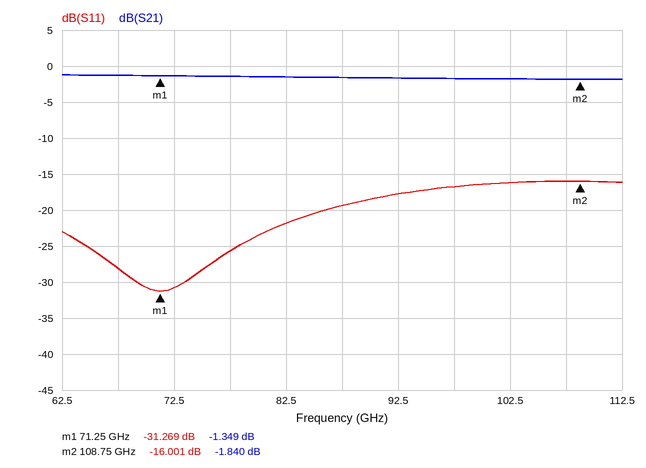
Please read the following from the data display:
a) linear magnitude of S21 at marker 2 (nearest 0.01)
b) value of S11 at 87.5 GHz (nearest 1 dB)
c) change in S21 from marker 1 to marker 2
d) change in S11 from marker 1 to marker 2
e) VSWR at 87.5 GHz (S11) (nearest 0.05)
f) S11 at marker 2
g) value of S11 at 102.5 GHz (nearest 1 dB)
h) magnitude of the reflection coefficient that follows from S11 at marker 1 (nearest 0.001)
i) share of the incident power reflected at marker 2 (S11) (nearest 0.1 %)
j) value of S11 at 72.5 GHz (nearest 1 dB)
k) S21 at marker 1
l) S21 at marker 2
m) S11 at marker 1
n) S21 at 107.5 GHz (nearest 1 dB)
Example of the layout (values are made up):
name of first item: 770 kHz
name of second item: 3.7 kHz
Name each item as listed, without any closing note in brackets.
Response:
linear magnitude of S21 at marker 2: 0.81
value of S11 at 87.5 GHz: -19 dB
change in S21 from marker 1 to marker 2: -0.491 dB
change in S11 from marker 1 to marker 2: 15.268 dB
VSWR at 87.5 GHz (S11): 1.25
S11 at marker 2: -16.001 dB
value of S11 at 102.5 GHz: -16 dB
magnitude of the reflection coefficient that follows from S11 at marker 1: 0.027
share of the incident power reflected at marker 2 (S11): 2.5 %
value of S11 at 72.5 GHz: -31 dB
S21 at marker 1: -1.349 dB
S21 at marker 2: -1.840 dB
S11 at marker 1: -31.269 dB
S21 at 107.5 GHz: -2 dB
